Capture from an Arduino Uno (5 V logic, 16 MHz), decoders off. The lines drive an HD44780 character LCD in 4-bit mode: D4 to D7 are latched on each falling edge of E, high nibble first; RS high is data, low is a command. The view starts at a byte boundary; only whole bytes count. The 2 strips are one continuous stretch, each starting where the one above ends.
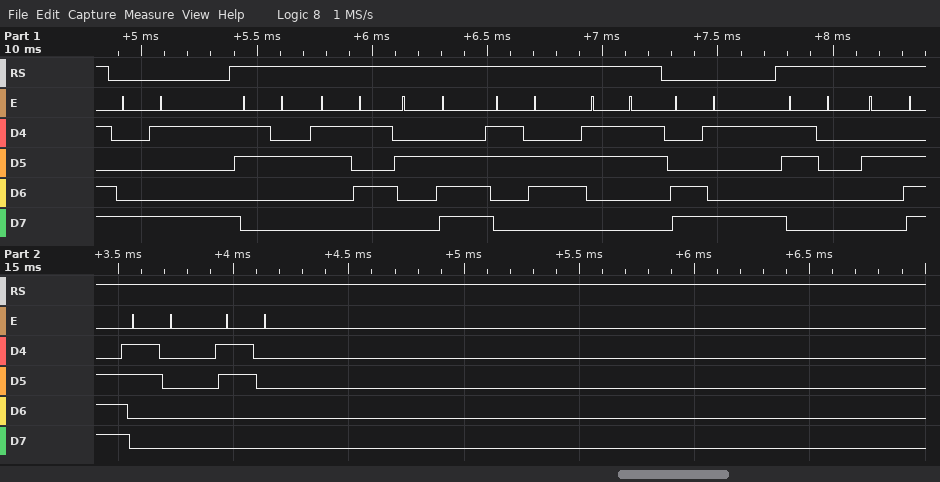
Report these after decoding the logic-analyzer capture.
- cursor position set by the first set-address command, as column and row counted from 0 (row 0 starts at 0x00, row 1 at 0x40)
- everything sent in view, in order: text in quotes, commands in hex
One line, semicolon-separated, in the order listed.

column 9, row 0; 0x89 "25.63" 0xC9 "0.00"
